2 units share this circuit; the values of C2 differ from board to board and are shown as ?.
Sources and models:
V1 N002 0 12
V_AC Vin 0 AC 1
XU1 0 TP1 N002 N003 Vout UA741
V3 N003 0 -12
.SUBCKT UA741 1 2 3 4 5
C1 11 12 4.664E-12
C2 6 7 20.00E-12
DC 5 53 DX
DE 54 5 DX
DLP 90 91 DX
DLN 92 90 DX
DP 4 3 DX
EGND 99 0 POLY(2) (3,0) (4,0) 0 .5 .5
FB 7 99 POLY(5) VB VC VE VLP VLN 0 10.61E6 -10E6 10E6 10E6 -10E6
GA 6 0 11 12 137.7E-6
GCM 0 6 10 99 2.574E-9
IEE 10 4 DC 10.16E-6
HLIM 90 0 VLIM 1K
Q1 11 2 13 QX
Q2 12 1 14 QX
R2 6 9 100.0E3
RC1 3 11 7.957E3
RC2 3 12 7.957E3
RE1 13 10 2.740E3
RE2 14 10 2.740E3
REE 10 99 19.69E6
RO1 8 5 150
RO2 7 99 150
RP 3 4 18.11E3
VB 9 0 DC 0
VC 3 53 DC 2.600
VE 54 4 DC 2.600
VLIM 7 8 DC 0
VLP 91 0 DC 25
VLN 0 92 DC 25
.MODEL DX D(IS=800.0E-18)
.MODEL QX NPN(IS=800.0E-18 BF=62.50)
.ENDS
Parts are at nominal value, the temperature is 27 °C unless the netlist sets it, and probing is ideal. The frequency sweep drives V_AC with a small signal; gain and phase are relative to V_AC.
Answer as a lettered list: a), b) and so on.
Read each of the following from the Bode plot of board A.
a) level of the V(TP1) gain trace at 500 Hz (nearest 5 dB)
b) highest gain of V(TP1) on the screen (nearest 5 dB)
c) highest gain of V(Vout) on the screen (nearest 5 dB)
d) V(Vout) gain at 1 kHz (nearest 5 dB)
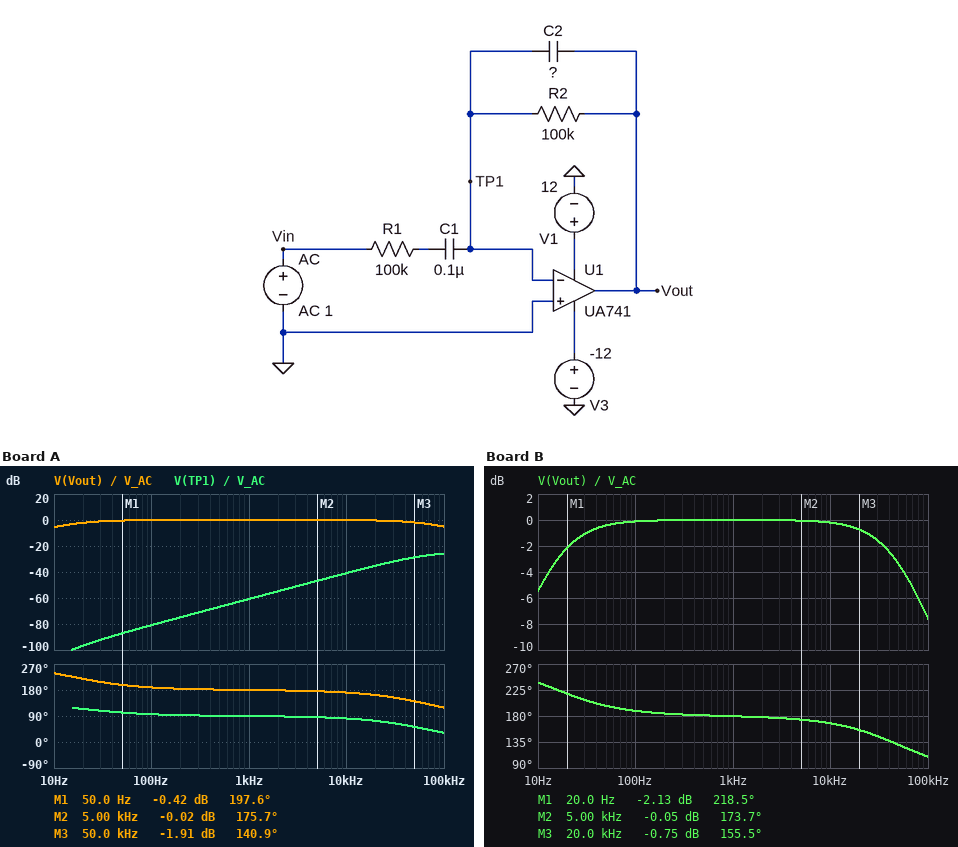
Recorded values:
a) -65 dB
b) -25 dB
c) 0 dB
d) 0 dB
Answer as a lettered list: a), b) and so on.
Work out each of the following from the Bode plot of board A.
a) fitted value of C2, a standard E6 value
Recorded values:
a) 22 pF
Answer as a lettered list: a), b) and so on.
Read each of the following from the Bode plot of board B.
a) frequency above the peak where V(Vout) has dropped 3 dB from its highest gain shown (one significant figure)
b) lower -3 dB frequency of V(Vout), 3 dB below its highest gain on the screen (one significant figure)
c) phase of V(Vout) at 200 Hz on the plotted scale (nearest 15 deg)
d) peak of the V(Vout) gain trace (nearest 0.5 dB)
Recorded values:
a) 50 kHz
b) 20 Hz
c) 180 deg
d) 0 dB
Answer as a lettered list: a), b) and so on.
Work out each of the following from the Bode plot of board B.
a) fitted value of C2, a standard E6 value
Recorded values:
a) 33 pF
